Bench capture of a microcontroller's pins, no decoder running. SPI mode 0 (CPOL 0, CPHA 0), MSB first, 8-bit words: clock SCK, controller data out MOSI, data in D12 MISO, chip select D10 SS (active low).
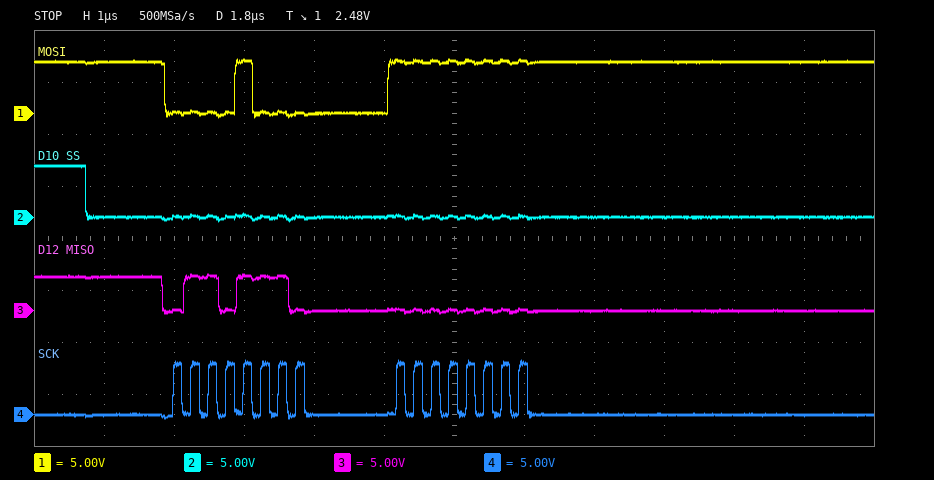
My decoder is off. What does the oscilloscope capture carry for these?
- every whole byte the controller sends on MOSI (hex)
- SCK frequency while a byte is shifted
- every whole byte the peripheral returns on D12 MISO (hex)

08 FF
4 MHz
6E 00
